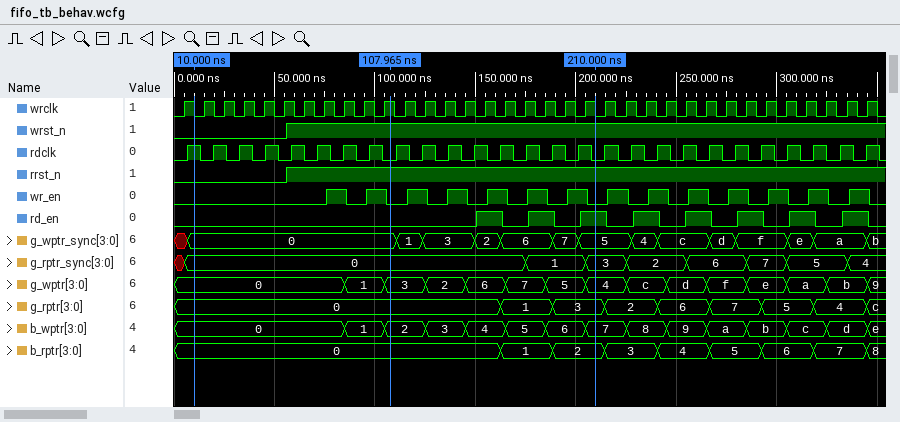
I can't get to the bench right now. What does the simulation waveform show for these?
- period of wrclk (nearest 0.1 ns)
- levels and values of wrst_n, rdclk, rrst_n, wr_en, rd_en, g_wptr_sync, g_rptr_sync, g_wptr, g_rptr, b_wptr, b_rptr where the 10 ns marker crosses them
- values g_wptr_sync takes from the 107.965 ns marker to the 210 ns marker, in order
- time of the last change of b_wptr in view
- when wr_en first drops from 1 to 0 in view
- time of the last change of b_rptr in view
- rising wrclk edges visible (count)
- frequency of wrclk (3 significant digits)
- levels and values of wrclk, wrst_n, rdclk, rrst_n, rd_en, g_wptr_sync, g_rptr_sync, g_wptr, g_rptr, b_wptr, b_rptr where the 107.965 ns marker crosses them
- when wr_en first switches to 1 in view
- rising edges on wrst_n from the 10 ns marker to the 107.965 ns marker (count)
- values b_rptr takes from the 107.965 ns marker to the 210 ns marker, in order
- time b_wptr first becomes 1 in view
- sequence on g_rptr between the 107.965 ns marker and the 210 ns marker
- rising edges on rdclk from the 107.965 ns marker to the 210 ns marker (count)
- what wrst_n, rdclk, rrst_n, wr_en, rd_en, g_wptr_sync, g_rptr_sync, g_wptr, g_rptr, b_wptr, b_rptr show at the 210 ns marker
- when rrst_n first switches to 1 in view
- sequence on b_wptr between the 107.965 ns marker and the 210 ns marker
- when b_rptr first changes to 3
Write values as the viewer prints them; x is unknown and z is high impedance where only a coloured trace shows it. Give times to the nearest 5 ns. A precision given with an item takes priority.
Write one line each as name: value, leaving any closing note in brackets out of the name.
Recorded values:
period of wrclk: 10 ns
levels and values of wrst_n, rdclk, rrst_n, wr_en, rd_en, g_wptr_sync, g_rptr_sync, g_wptr, g_rptr, b_wptr, b_rptr where the 10 ns marker crosses them: wrst_n=0, rdclk=1, rrst_n=0, wr_en=0, rd_en=0, g_wptr_sync=0, g_rptr_sync=0, g_wptr=0, g_rptr=0, b_wptr=0, b_rptr=0
values g_wptr_sync takes from the 107.965 ns marker to the 210 ns marker, in order: 0, 1, 3, 2, 6, 7, 5
time of the last change of b_wptr in view: 345 ns
when wr_en first drops from 1 to 0 in view: 85 ns
time of the last change of b_rptr in view: 345 ns
rising wrclk edges visible: 35
frequency of wrclk: 100 MHz
levels and values of wrclk, wrst_n, rdclk, rrst_n, rd_en, g_wptr_sync, g_rptr_sync, g_wptr, g_rptr, b_wptr, b_rptr where the 107.965 ns marker crosses them: wrclk=1, wrst_n=1, rdclk=0, rrst_n=1, rd_en=0, g_wptr_sync=0, g_rptr_sync=0, g_wptr=3, g_rptr=0, b_wptr=2, b_rptr=0
when wr_en first switches to 1 in view: 75 ns
rising edges on wrst_n from the 10 ns marker to the 107.965 ns marker: 1
values b_rptr takes from the 107.965 ns marker to the 210 ns marker, in order: 0, 1, 2
time b_wptr first becomes 1 in view: 85 ns
sequence on g_rptr between the 107.965 ns marker and the 210 ns marker: 0, 1, 3
rising edges on rdclk from the 107.965 ns marker to the 210 ns marker: 8
what wrst_n, rdclk, rrst_n, wr_en, rd_en, g_wptr_sync, g_rptr_sync, g_wptr, g_rptr, b_wptr, b_rptr show at the 210 ns marker: wrst_n=1, rdclk=0, rrst_n=1, wr_en=0, rd_en=1, g_wptr_sync=5, g_rptr_sync=3, g_wptr=4, g_rptr=3, b_wptr=7, b_rptr=2
when rrst_n first switches to 1 in view: 55 ns
sequence on b_wptr between the 107.965 ns marker and the 210 ns marker: 2, 3, 4, 5, 6, 7
when b_rptr first changes to 3: 215 ns
